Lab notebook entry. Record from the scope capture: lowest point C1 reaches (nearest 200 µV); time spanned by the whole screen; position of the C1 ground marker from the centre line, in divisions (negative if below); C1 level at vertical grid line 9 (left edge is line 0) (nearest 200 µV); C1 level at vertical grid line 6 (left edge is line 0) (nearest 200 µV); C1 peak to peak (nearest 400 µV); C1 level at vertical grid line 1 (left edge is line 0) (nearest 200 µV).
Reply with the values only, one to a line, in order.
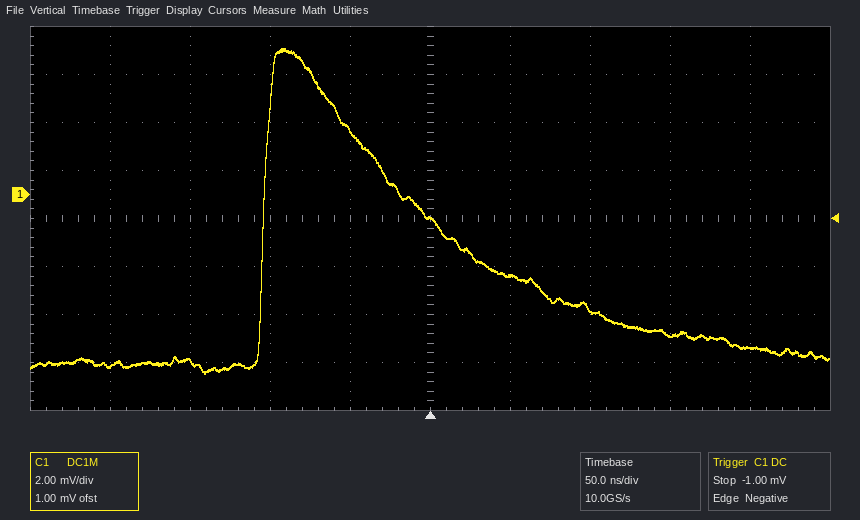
-7.4 mV
500 ns
+0.5 div
-6.4 mV
-3.4 mV
13.6 mV
-7.2 mV
